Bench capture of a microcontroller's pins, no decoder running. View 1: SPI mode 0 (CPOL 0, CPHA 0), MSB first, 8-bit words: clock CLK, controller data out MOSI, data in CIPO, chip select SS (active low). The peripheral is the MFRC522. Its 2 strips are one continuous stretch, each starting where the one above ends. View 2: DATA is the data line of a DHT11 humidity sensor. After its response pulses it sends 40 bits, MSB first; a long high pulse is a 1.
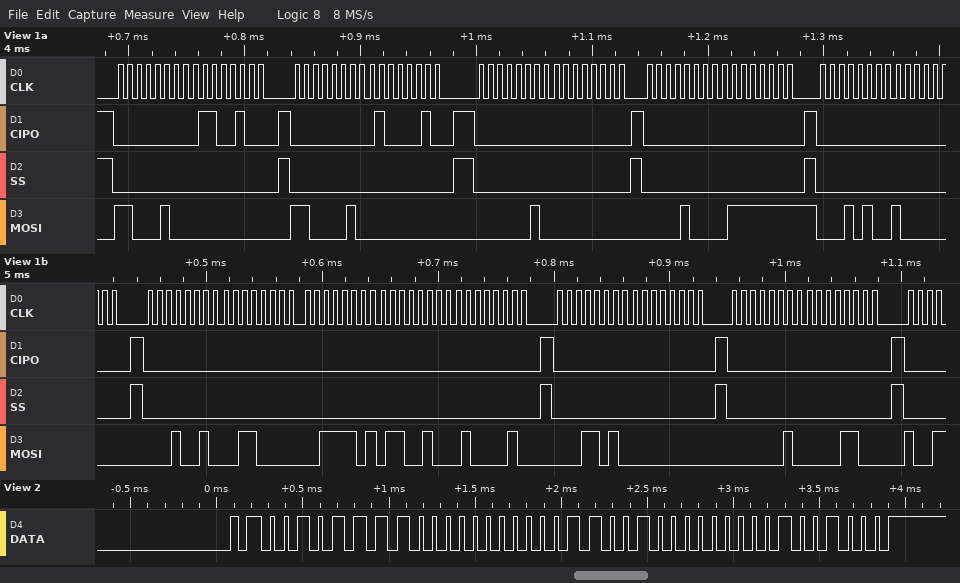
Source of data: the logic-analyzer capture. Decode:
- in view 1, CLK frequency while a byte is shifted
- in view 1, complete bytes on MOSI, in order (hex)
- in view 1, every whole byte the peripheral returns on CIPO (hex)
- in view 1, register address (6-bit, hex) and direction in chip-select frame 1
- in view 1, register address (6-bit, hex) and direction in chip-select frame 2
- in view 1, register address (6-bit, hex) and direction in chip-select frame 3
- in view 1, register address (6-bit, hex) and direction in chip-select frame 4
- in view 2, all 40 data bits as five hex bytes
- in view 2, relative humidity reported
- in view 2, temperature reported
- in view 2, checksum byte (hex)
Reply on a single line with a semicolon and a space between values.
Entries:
125 kHz; C4 00 C2 00 02 00 08 7F 14 80 12 30 3D 64 42 1A 00 02 0C; 00 64 00 42 00 00 00 00 00 00 00 00 00 00 00 00 00 00 00; 0x22 read; 0x21 read; 0x01 write; 0x04 write; 2F 00 19 00 48; 47 %; 25.0 °C; 0x48
